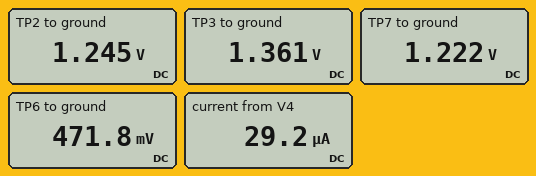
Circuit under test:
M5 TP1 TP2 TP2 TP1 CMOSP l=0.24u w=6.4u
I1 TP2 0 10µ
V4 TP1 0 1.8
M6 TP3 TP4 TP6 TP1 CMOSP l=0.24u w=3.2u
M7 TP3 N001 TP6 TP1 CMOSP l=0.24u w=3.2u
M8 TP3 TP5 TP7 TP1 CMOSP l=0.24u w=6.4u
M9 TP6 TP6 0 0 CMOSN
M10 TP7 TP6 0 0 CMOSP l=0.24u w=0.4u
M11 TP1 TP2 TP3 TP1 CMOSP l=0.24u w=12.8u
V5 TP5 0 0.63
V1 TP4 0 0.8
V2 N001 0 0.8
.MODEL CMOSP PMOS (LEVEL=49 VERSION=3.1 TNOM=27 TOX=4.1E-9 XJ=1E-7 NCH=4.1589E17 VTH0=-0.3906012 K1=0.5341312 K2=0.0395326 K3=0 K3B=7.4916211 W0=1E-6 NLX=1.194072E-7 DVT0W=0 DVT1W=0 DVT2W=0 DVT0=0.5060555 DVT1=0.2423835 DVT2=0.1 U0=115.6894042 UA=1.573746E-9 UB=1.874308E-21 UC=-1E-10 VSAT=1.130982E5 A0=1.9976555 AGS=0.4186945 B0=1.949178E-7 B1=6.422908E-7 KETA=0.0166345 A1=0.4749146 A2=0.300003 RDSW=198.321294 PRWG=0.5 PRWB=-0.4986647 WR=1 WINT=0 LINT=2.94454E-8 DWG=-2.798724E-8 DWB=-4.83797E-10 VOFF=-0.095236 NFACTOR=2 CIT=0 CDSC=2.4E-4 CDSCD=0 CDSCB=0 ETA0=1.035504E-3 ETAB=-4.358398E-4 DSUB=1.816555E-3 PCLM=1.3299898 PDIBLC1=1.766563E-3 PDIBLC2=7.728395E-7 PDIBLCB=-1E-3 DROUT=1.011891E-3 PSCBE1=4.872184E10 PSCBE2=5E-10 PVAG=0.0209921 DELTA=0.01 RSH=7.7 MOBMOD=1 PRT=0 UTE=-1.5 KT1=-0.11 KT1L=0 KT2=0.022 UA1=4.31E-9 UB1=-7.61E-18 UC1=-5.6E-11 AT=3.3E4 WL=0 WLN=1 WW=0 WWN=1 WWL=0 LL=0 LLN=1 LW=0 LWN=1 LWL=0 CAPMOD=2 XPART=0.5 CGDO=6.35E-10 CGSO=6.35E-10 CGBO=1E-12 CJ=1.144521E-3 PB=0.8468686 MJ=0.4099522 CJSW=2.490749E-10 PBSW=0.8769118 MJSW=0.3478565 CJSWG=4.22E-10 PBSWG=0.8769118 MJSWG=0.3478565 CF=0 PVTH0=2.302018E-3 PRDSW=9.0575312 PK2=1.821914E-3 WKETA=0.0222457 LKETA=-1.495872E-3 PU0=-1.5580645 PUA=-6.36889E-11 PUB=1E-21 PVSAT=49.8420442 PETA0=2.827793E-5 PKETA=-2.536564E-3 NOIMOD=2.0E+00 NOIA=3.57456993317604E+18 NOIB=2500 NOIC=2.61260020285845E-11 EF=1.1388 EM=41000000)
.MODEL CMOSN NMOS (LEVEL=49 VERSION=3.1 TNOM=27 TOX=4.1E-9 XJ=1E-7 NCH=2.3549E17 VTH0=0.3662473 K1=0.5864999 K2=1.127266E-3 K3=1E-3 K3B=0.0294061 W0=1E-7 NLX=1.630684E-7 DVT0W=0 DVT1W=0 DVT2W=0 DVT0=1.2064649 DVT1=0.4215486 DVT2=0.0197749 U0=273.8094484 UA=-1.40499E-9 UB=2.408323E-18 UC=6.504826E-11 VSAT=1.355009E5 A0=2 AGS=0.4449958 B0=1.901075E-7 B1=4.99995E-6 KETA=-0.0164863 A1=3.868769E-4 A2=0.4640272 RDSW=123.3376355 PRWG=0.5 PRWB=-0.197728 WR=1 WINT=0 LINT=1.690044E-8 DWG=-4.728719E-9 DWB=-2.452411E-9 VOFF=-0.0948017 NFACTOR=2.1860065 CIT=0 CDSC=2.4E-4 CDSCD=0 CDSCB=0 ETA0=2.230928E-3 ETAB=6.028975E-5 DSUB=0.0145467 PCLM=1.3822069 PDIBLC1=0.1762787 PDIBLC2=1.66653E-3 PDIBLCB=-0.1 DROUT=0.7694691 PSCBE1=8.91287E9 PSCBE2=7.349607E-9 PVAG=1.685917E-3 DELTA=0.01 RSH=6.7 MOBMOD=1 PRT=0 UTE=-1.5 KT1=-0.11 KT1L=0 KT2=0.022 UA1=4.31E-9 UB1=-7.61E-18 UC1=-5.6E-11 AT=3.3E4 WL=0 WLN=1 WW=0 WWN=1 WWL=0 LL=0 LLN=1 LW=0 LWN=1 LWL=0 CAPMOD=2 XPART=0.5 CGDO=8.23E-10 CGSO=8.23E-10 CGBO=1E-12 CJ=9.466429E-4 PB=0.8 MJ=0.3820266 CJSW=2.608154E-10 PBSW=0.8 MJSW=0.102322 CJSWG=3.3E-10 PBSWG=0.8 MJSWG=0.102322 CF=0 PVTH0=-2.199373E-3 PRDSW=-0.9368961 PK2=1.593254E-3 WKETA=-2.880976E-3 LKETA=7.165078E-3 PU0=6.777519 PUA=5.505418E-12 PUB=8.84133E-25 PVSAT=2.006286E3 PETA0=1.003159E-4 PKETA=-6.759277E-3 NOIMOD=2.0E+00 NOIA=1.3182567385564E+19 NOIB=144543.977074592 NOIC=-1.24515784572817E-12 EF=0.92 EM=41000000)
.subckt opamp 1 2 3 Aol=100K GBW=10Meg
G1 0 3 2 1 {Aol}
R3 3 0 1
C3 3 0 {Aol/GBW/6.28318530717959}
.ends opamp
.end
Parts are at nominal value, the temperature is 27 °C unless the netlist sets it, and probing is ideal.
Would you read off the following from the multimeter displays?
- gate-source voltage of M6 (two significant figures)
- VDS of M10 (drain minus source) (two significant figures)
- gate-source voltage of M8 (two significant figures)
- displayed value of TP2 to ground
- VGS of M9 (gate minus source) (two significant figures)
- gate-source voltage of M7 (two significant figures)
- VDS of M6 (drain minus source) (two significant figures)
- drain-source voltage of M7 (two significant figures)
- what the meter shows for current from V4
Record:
330 mV
1.2 V
-590 mV
1.245 V
470 mV
330 mV
890 mV
890 mV
29.2 µA
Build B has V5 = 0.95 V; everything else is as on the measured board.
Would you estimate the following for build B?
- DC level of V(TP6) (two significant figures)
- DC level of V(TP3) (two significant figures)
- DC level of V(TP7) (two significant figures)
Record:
780 mV
1.5 V
1.1 V
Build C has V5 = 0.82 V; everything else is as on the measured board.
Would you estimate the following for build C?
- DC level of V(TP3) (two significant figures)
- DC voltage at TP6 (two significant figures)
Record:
1.5 V
700 mV
